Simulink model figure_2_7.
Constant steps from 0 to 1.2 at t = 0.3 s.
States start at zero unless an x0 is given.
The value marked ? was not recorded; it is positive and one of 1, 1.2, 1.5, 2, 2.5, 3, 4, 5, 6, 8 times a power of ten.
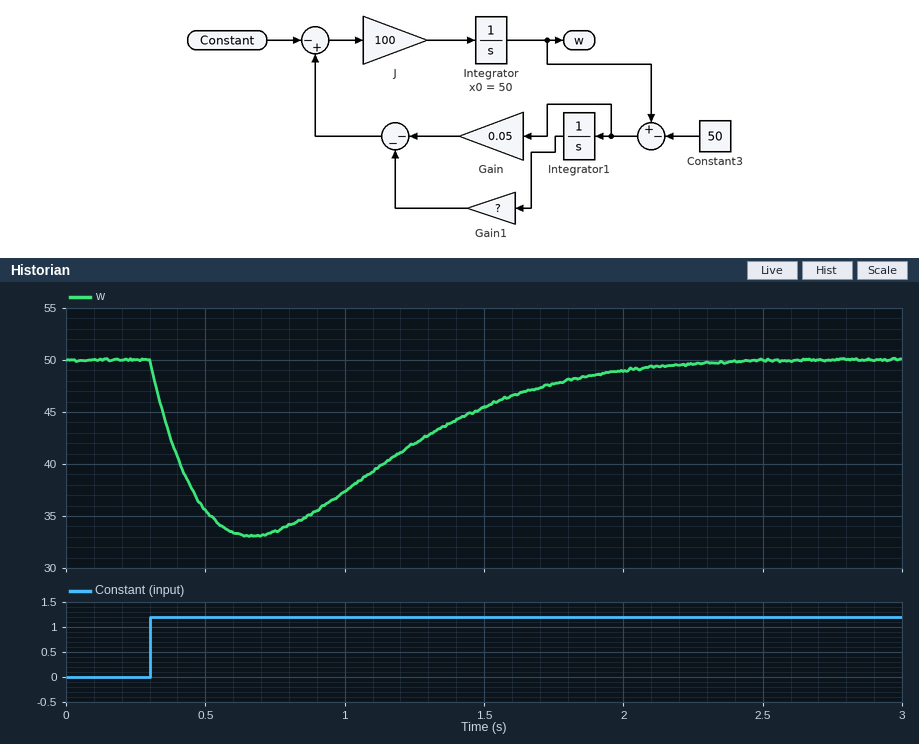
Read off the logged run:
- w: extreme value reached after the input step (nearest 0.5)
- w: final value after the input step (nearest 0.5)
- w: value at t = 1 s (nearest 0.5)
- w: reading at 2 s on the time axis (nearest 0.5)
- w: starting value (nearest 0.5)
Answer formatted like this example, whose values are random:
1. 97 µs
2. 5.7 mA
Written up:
1. 33.0
2. 50.0
3. 37.5
4. 49.0
5. 50.0
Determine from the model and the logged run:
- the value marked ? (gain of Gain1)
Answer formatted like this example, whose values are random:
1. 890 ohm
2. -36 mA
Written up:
1. 0.08
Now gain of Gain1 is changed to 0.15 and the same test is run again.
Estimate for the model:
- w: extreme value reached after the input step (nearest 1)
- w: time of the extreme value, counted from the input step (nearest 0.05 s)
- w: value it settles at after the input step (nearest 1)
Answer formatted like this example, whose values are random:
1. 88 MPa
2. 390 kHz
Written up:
1. 35
2. 0.30 s
3. 50
